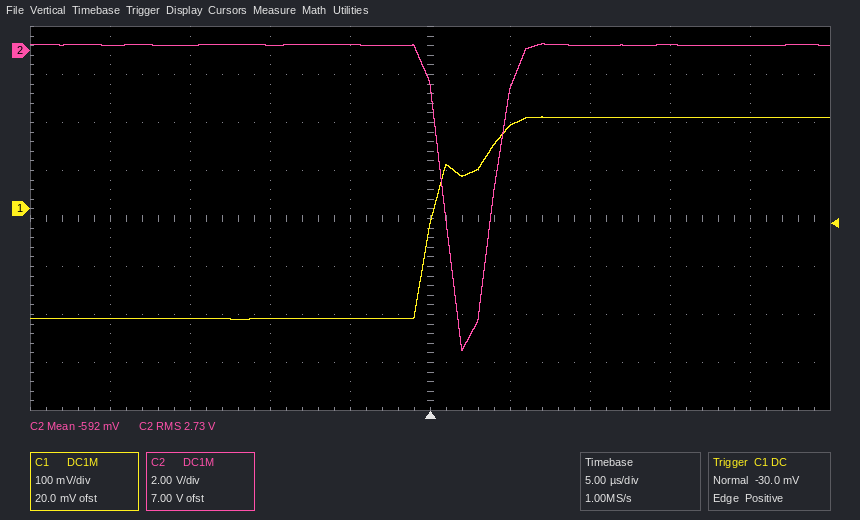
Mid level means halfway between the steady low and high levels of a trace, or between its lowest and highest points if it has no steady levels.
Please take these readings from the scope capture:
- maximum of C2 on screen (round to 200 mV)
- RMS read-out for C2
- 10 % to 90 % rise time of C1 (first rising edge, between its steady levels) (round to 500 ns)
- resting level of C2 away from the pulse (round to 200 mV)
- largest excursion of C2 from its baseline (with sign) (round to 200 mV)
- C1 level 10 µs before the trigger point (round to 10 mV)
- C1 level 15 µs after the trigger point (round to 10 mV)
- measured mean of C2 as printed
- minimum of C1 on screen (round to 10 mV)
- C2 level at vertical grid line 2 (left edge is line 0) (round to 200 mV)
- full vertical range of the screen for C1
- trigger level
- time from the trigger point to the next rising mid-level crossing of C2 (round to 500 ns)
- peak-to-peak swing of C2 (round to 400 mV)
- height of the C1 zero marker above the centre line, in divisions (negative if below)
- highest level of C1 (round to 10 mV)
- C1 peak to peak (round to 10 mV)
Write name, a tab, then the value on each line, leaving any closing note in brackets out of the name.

maximum of C2 on screen	200 mV
RMS read-out for C2	2.73 V
10 % to 90 % rise time of C1 (first rising edge, between its steady levels)	5.0 µs
resting level of C2 away from the pulse	200 mV
largest excursion of C2 from its baseline (with sign)	-12.8 V
C1 level 10 µs before the trigger point	-230 mV
C1 level 15 µs after the trigger point	190 mV
measured mean of C2 as printed	-592 mV
minimum of C1 on screen	-230 mV
C2 level at vertical grid line 2 (left edge is line 0)	200 mV
full vertical range of the screen for C1	800 mV
trigger level	-30.0 mV
time from the trigger point to the next rising mid-level crossing of C2	4.0 µs
peak-to-peak swing of C2	12.8 V
height of the C1 zero marker above the centre line, in divisions	+0.2 div
highest level of C1	190 mV
C1 peak to peak	420 mV
